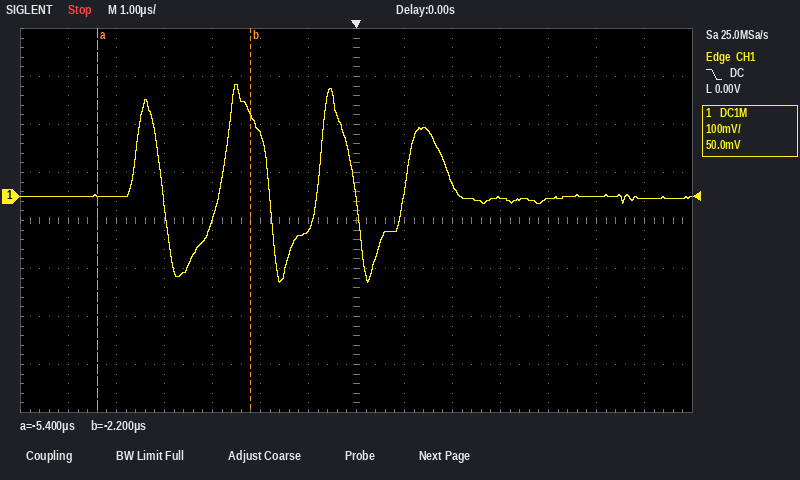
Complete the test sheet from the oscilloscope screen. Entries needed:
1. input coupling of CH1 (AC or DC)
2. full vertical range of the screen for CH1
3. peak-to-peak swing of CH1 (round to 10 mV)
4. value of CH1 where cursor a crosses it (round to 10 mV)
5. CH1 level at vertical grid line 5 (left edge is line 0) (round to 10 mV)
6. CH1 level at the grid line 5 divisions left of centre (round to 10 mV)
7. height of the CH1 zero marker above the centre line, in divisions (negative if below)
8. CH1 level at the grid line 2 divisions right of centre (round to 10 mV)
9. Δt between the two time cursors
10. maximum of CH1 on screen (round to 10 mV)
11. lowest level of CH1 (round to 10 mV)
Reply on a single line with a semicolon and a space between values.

DC; 800 mV; 410 mV; 0 mV; 130 mV; 0 mV; +0.5 div; 30 mV; 3.2 µs; 230 mV; -180 mV
